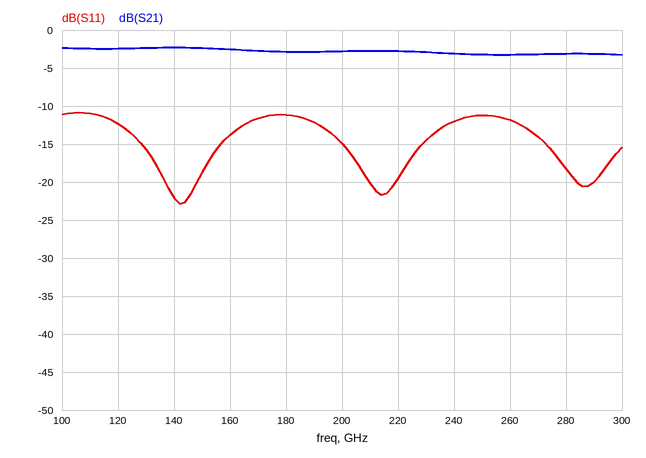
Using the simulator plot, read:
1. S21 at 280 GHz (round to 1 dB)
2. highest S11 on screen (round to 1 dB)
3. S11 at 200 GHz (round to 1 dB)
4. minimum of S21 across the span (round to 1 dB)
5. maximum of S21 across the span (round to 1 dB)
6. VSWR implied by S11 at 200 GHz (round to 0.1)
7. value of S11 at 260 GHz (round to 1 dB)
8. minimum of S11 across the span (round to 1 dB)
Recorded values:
-3 dB
-11 dB
-15 dB
-3 dB
-2 dB
1.4
-12 dB
-23 dB
